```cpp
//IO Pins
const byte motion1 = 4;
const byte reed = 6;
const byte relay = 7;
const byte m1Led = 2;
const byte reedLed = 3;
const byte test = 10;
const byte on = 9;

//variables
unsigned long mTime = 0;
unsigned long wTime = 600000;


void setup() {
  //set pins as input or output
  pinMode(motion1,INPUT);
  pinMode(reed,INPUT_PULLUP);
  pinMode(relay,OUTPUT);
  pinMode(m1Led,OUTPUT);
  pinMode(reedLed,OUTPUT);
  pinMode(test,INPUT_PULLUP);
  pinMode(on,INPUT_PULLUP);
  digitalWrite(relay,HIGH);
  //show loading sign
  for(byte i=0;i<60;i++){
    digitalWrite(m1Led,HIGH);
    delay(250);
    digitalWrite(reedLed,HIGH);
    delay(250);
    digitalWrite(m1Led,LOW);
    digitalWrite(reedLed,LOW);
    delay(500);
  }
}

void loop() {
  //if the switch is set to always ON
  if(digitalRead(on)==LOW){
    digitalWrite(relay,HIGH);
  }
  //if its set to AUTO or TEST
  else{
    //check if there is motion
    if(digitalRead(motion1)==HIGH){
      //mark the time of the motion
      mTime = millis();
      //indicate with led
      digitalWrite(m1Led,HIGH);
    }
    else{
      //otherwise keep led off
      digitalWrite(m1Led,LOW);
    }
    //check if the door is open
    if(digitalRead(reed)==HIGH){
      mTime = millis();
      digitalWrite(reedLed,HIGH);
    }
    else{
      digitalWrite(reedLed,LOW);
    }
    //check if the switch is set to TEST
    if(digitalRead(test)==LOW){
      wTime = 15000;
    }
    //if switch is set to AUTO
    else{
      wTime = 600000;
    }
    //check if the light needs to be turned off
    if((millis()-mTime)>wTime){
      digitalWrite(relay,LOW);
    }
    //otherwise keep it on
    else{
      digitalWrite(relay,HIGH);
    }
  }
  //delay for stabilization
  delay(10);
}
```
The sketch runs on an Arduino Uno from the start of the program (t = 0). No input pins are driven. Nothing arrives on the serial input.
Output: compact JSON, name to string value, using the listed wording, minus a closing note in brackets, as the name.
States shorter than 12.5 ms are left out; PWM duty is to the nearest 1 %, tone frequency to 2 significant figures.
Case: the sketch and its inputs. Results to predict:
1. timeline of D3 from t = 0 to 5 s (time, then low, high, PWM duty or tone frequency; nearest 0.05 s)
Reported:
{"timeline of D3 from t = 0 to 5 s": "0 s low; 0.25 s high; 0.5 s low; 1.25 s high; 1.5 s low; 2.25 s high; 2.5 s low; 3.25 s high; 3.5 s low; 4.25 s high; 4.5 s low"}
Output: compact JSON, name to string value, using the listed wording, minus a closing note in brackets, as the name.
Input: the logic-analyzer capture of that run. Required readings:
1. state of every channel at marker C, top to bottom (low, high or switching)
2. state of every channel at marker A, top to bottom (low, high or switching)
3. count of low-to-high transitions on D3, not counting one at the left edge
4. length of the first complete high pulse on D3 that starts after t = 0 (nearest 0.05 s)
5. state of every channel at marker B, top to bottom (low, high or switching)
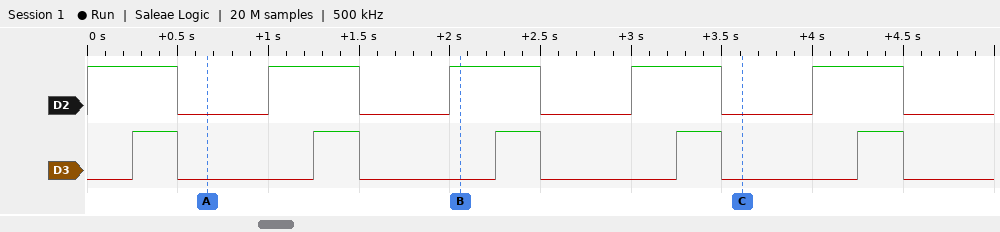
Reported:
{"state of every channel at marker C, top to bottom": "D2 low, D3 low", "state of every channel at marker A, top to bottom": "D2 low, D3 low", "count of low-to-high transitions on D3, not counting one at the left edge": "5", "length of the first complete high pulse on D3 that starts after t = 0": "0.25 s", "state of every channel at marker B, top to bottom": "D2 high, D3 low"}
